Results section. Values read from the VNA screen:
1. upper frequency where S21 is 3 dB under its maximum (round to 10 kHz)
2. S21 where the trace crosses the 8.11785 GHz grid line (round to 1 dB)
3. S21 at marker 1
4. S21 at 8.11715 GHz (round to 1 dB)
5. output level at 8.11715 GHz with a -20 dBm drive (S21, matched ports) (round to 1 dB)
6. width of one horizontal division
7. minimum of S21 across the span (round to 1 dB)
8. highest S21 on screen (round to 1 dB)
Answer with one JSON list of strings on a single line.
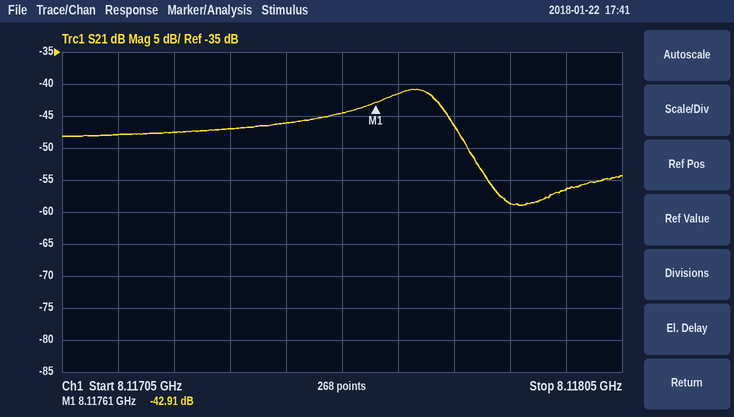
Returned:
["8.11773 GHz", "-59 dB", "-42.91 dB", "-48 dB", "-68 dBm", "100 kHz", "-59 dB", "-41 dB"]
